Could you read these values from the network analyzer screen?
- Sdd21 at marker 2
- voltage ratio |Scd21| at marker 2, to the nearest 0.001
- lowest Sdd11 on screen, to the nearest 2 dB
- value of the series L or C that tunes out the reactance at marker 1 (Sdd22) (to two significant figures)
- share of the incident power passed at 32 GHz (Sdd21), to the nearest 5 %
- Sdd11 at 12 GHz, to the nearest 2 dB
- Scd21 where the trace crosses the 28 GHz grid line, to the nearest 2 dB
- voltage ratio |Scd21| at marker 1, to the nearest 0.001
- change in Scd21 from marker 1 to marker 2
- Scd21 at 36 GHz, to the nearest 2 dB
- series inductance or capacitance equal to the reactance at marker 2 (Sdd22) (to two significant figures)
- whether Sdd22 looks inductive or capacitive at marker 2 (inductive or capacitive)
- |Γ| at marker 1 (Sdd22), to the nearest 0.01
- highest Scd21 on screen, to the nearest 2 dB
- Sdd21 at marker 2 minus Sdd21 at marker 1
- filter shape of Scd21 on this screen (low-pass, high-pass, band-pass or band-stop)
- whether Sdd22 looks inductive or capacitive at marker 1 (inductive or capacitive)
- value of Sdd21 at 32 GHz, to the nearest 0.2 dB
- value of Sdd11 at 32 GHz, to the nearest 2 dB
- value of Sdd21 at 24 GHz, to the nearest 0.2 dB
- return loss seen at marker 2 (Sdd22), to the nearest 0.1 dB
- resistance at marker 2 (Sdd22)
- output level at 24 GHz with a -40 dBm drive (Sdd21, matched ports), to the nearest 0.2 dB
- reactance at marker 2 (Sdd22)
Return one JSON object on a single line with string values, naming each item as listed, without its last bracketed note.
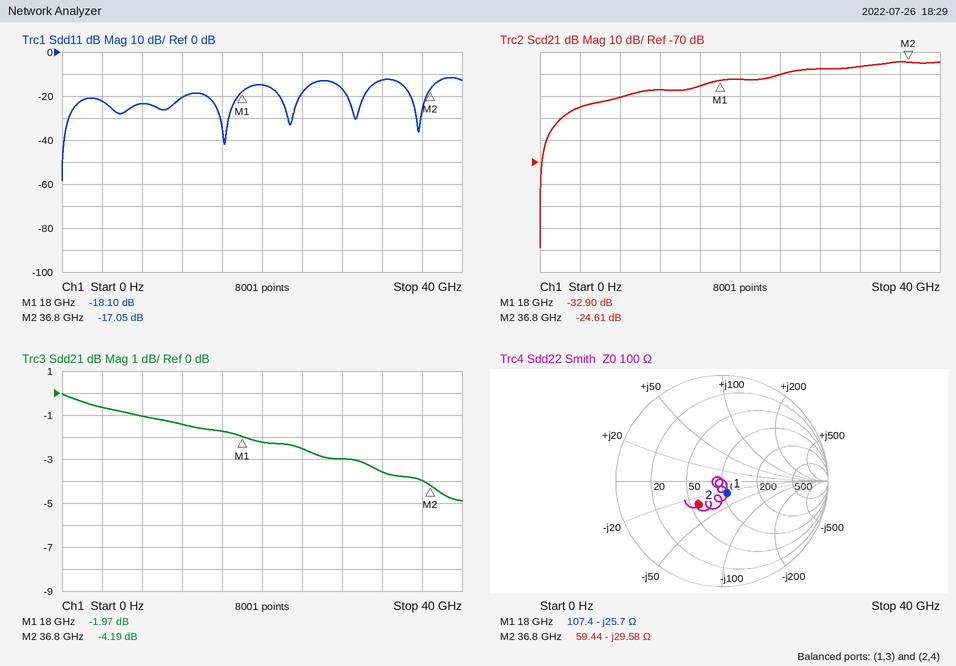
{"Sdd21 at marker 2": "-4.19 dB", "voltage ratio |Scd21| at marker 2, to the nearest 0.001": "0.059", "lowest Sdd11 on screen, to the nearest 2 dB": "-58 dB", "value of the series L or C that tunes out the reactance at marker 1 (Sdd22)": "230 pH", "share of the incident power passed at 32 GHz (Sdd21), to the nearest 5 %": "45 %", "Sdd11 at 12 GHz, to the nearest 2 dB": "-20 dB", "Scd21 where the trace crosses the 28 GHz grid line, to the nearest 2 dB": "-28 dB", "voltage ratio |Scd21| at marker 1, to the nearest 0.001": "0.023", "change in Scd21 from marker 1 to marker 2": "8.29 dB", "Scd21 at 36 GHz, to the nearest 2 dB": "-24 dB", "series inductance or capacitance equal to the reactance at marker 2 (Sdd22)": "150 fF", "whether Sdd22 looks inductive or capacitive at marker 2": "capacitive", "|Γ| at marker 1 (Sdd22), to the nearest 0.01": "0.13", "highest Scd21 on screen, to the nearest 2 dB": "-24 dB", "Sdd21 at marker 2 minus Sdd21 at marker 1": "-2.22 dB", "filter shape of Scd21 on this screen": "high-pass", "whether Sdd22 looks inductive or capacitive at marker 1": "capacitive", "value of Sdd21 at 32 GHz, to the nearest 0.2 dB": "-3.6 dB", "value of Sdd11 at 32 GHz, to the nearest 2 dB": "-12 dB", "value of Sdd21 at 24 GHz, to the nearest 0.2 dB": "-2.6 dB", "return loss seen at marker 2 (Sdd22), to the nearest 0.1 dB": "10.2 dB", "resistance at marker 2": "59.44 Ω", "output level at 24 GHz with a -40 dBm drive (Sdd21, matched ports), to the nearest 0.2 dB": "-42.6 dBm", "reactance at marker 2": "-29.58 Ω"}
